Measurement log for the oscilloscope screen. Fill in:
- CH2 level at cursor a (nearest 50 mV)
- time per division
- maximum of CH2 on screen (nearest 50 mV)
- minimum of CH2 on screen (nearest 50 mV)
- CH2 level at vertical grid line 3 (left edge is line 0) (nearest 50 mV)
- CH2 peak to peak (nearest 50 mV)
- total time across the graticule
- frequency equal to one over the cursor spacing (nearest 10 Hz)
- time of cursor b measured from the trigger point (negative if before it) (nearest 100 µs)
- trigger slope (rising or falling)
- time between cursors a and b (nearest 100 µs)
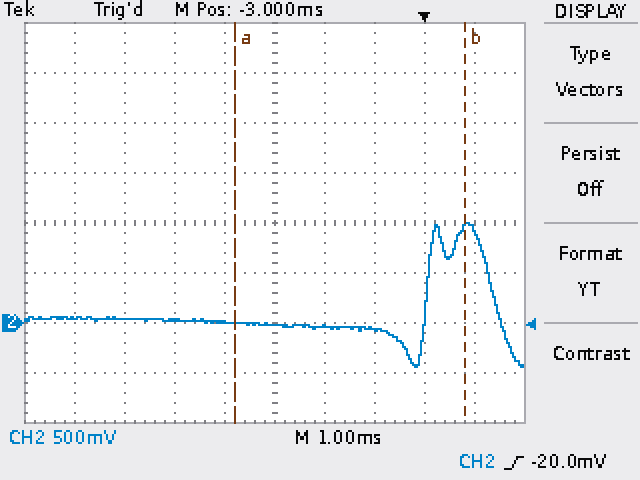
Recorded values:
0 mV
1 ms
1.00 V
-450 mV
50 mV
1.45 V
10 ms
220 Hz
+800 µs
rising
4.6 ms
